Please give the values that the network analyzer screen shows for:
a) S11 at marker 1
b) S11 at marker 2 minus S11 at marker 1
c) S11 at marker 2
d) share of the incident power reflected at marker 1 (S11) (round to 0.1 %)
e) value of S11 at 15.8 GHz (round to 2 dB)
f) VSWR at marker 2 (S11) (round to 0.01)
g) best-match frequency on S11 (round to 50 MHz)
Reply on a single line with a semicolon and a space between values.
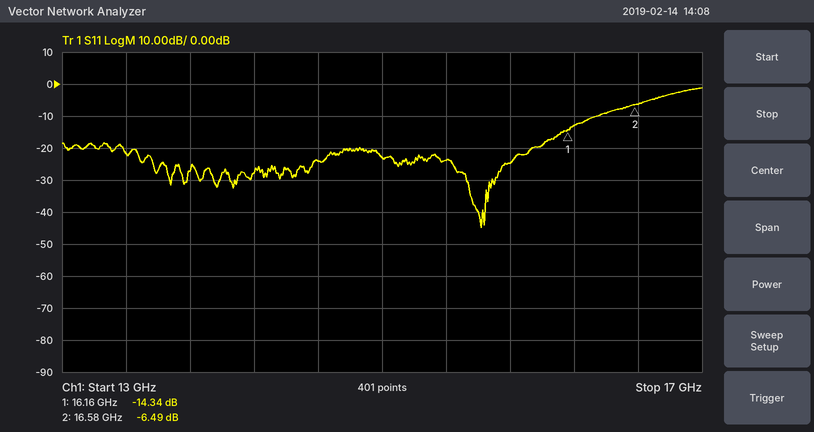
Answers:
-14.34 dB; 7.85 dB; -6.49 dB; 3.7 %; -24 dB; 2.80; 15.60 GHz
